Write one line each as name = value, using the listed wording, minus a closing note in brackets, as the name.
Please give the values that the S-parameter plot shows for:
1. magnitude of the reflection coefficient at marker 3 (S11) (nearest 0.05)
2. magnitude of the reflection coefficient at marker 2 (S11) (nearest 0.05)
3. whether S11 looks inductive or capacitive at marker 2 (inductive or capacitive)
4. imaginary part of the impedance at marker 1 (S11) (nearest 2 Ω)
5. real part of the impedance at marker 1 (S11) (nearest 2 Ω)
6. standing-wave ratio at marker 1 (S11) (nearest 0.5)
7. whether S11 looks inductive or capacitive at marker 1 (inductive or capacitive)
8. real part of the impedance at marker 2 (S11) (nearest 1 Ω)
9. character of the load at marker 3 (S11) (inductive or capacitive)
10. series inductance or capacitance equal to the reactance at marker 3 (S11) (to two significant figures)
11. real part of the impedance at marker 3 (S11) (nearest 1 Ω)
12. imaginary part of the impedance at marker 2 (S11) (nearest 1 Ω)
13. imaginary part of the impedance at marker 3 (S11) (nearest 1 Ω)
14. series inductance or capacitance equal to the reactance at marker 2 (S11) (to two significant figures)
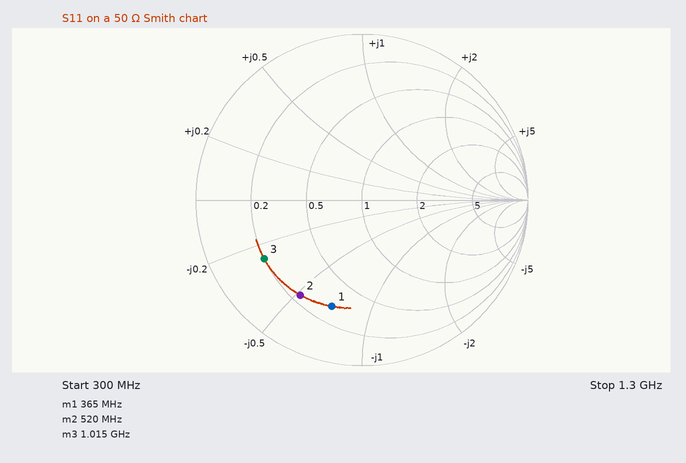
magnitude of the reflection coefficient at marker 3 (S11) = 0.70
magnitude of the reflection coefficient at marker 2 (S11) = 0.70
whether S11 looks inductive or capacitive at marker 2 = capacitive
imaginary part of the impedance at marker 1 (S11) = -36 Ω
real part of the impedance at marker 1 (S11) = 16 Ω
standing-wave ratio at marker 1 (S11) = 5.0
whether S11 looks inductive or capacitive at marker 1 = capacitive
real part of the impedance at marker 2 (S11) = 12 Ω
character of the load at marker 3 (S11) = capacitive
series inductance or capacitance equal to the reactance at marker 3 (S11) = 12 pF
real part of the impedance at marker 3 (S11) = 10 Ω
imaginary part of the impedance at marker 2 (S11) = -26 Ω
imaginary part of the impedance at marker 3 (S11) = -13 Ω
series inductance or capacitance equal to the reactance at marker 2 (S11) = 12 pF
